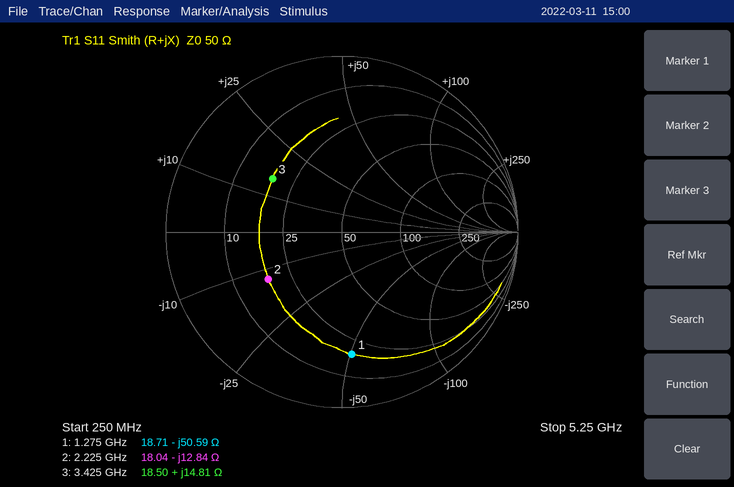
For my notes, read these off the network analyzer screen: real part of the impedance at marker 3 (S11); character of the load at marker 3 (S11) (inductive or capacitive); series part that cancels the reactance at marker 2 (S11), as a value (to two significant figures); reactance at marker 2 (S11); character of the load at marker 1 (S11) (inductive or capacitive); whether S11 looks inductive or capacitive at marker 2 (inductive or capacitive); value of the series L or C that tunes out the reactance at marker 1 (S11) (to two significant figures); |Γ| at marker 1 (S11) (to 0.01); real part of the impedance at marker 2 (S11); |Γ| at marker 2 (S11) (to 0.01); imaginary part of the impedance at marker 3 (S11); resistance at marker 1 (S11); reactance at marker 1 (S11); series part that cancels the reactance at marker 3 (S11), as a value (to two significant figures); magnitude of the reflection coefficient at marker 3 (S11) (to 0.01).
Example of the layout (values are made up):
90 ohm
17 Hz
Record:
18.50 Ω
inductive
920 pH
-12.84 Ω
capacitive
capacitive
6.3 nH
0.70
18.04 Ω
0.50
+14.81 Ω
18.71 Ω
-50.59 Ω
3.1 pF
0.50
